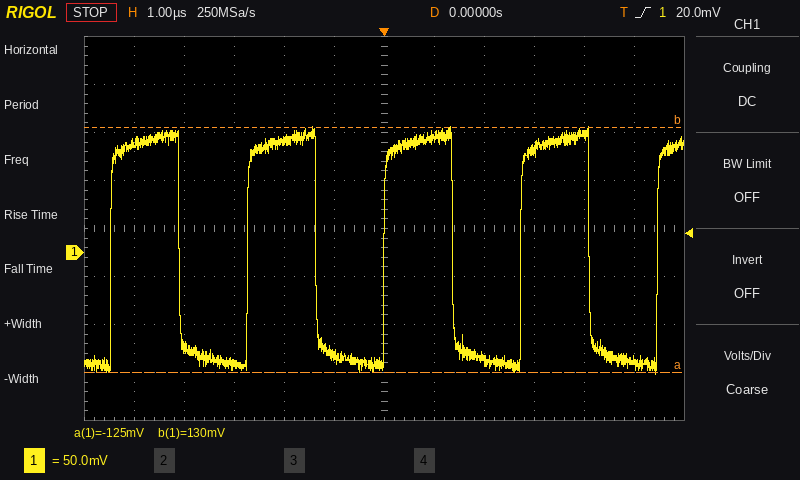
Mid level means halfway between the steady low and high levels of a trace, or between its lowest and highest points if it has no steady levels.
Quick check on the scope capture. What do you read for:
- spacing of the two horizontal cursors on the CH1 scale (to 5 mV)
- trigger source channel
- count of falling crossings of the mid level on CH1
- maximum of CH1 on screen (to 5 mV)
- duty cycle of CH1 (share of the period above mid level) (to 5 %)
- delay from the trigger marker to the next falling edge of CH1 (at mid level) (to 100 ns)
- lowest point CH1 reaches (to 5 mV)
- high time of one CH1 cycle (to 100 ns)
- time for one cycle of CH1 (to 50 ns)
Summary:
255 mV
CH1
4
130 mV
50 %
1.4 µs
-125 mV
1.4 µs
2.75 µs
